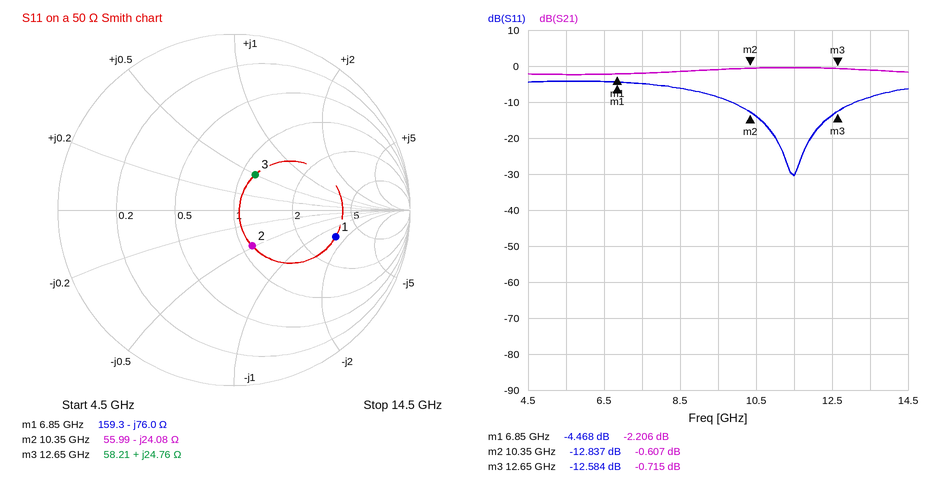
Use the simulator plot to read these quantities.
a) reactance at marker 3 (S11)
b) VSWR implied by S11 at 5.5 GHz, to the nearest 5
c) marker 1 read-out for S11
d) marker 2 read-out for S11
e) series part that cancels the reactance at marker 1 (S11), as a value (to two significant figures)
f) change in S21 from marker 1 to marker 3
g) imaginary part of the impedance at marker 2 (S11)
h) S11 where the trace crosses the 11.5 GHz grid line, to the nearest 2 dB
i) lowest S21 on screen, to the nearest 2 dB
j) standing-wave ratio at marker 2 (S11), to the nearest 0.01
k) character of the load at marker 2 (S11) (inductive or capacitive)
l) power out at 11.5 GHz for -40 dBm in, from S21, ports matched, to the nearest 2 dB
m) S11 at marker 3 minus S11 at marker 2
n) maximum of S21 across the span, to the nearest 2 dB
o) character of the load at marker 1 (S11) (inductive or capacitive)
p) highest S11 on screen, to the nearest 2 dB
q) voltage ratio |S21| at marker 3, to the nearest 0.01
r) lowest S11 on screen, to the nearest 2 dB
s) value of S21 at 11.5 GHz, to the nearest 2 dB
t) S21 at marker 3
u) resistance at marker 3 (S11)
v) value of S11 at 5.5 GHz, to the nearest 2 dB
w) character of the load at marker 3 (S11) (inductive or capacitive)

+24.76 Ω
5
-4.468 dB
-12.837 dB
1.8 nH
1.491 dB
-24.08 Ω
-30 dB
-2 dB
1.59
capacitive
-40 dBm
0.253 dB
0 dB
capacitive
-4 dB
0.92
-30 dB
0 dB
-0.715 dB
58.21 Ω
-4 dB
inductive
